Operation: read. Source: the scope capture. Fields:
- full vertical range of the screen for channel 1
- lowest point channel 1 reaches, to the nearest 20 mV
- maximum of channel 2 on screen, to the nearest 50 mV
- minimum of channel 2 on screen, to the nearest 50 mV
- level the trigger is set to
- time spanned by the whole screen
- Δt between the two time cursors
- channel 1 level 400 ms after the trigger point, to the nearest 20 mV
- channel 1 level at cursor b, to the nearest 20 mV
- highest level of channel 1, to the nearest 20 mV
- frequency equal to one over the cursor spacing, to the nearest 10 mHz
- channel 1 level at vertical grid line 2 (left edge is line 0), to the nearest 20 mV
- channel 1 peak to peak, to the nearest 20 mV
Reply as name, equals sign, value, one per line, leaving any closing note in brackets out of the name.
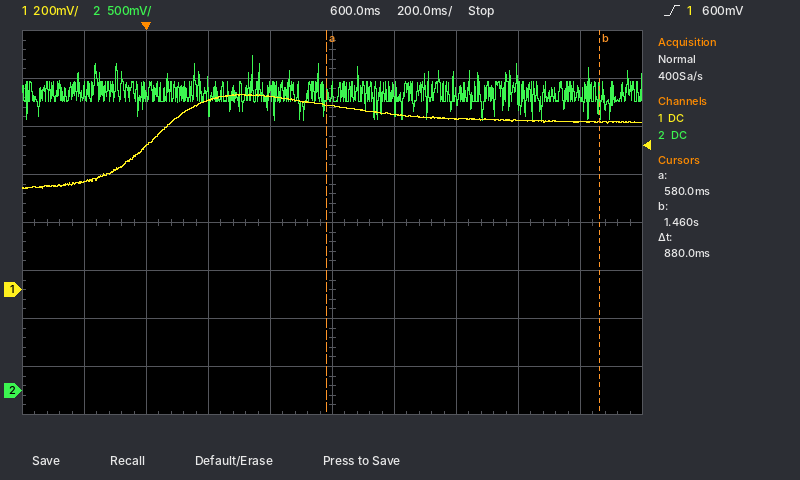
full vertical range of the screen for channel 1 = 1.6 V
lowest point channel 1 reaches, to the nearest 20 mV = 420 mV
maximum of channel 2 on screen, to the nearest 50 mV = 3.50 V
minimum of channel 2 on screen, to the nearest 50 mV = 2.80 V
level the trigger is set to = 600 mV
time spanned by the whole screen = 2 s
Δt between the two time cursors = 880 ms
channel 1 level 400 ms after the trigger point, to the nearest 20 mV = 800 mV
channel 1 level at cursor b, to the nearest 20 mV = 700 mV
highest level of channel 1, to the nearest 20 mV = 820 mV
frequency equal to one over the cursor spacing, to the nearest 10 mHz = 1.14 Hz
channel 1 level at vertical grid line 2 (left edge is line 0), to the nearest 20 mV = 600 mV
channel 1 peak to peak, to the nearest 20 mV = 400 mV
